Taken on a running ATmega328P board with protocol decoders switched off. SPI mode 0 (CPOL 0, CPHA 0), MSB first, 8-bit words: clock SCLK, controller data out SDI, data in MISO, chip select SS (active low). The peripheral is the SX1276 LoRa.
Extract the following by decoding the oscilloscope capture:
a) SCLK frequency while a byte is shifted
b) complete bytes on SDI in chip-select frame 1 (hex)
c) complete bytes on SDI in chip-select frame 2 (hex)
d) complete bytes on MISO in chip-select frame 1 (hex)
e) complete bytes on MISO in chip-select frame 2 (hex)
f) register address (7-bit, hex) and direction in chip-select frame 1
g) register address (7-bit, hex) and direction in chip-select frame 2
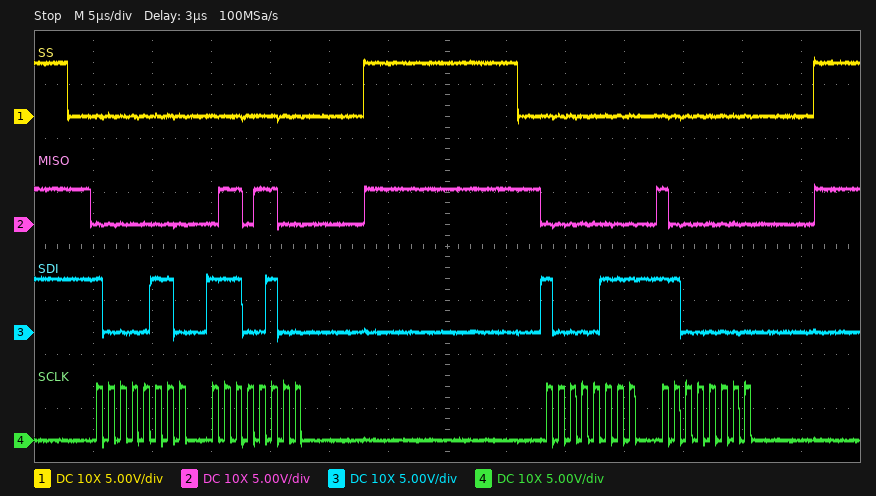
1 MHz
0x86 0xE4
0x87 0xC0
0x00 0x6C
0x00 0x80
0x06 write
0x07 write
